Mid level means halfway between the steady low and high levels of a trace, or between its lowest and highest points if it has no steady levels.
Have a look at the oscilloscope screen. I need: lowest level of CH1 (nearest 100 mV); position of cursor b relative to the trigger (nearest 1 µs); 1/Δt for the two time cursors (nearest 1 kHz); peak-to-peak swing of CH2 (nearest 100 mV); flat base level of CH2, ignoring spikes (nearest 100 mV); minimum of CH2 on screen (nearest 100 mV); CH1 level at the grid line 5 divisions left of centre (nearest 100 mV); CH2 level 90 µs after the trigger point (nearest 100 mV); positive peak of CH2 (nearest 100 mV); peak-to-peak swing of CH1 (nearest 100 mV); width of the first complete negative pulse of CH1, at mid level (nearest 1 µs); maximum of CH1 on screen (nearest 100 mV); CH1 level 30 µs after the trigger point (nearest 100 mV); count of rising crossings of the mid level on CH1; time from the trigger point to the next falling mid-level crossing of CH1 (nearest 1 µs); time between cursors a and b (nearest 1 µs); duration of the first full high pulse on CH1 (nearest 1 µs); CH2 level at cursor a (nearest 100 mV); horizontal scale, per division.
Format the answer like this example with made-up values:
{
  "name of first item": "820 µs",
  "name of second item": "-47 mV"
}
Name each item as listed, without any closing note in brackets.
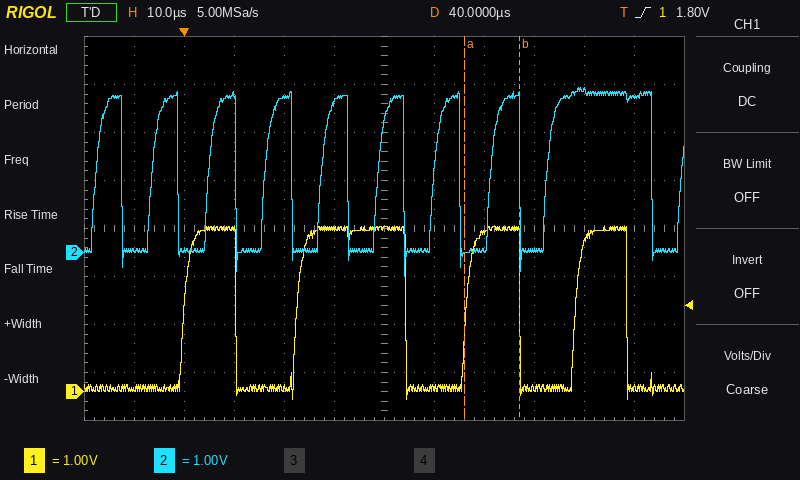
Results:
{
  "lowest level of CH1": "-200 mV",
  "position of cursor b relative to the trigger": "+67 µs",
  "1/Δt for the two time cursors": "91 kHz",
  "peak-to-peak swing of CH2": "3.9 V",
  "flat base level of CH2, ignoring spikes": "0.0 V",
  "minimum of CH2 on screen": "-500 mV",
  "CH1 level at the grid line 5 divisions left of centre": "100 mV",
  "CH2 level 90 µs after the trigger point": "3.2 V",
  "positive peak of CH2": "3.4 V",
  "peak-to-peak swing of CH1": "3.6 V",
  "width of the first complete negative pulse of CH1, at mid level": "12 µs",
  "maximum of CH1 on screen": "3.4 V",
  "CH1 level 30 µs after the trigger point": "3.4 V",
  "count of rising crossings of the mid level on CH1": "4",
  "time from the trigger point to the next falling mid-level crossing of CH1": "10 µs",
  "time between cursors a and b": "11 µs",
  "duration of the first full high pulse on CH1": "10 µs",
  "CH2 level at cursor a": "0.0 V",
  "horizontal scale, per division": "10 µs"
}
